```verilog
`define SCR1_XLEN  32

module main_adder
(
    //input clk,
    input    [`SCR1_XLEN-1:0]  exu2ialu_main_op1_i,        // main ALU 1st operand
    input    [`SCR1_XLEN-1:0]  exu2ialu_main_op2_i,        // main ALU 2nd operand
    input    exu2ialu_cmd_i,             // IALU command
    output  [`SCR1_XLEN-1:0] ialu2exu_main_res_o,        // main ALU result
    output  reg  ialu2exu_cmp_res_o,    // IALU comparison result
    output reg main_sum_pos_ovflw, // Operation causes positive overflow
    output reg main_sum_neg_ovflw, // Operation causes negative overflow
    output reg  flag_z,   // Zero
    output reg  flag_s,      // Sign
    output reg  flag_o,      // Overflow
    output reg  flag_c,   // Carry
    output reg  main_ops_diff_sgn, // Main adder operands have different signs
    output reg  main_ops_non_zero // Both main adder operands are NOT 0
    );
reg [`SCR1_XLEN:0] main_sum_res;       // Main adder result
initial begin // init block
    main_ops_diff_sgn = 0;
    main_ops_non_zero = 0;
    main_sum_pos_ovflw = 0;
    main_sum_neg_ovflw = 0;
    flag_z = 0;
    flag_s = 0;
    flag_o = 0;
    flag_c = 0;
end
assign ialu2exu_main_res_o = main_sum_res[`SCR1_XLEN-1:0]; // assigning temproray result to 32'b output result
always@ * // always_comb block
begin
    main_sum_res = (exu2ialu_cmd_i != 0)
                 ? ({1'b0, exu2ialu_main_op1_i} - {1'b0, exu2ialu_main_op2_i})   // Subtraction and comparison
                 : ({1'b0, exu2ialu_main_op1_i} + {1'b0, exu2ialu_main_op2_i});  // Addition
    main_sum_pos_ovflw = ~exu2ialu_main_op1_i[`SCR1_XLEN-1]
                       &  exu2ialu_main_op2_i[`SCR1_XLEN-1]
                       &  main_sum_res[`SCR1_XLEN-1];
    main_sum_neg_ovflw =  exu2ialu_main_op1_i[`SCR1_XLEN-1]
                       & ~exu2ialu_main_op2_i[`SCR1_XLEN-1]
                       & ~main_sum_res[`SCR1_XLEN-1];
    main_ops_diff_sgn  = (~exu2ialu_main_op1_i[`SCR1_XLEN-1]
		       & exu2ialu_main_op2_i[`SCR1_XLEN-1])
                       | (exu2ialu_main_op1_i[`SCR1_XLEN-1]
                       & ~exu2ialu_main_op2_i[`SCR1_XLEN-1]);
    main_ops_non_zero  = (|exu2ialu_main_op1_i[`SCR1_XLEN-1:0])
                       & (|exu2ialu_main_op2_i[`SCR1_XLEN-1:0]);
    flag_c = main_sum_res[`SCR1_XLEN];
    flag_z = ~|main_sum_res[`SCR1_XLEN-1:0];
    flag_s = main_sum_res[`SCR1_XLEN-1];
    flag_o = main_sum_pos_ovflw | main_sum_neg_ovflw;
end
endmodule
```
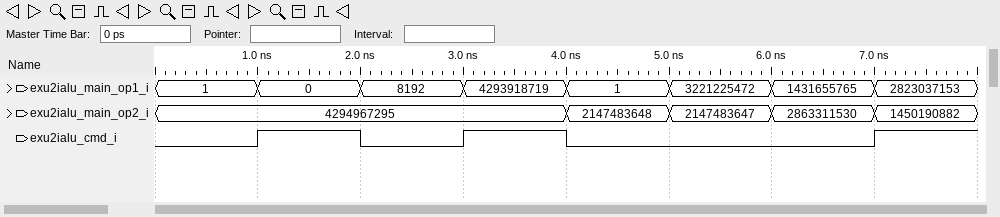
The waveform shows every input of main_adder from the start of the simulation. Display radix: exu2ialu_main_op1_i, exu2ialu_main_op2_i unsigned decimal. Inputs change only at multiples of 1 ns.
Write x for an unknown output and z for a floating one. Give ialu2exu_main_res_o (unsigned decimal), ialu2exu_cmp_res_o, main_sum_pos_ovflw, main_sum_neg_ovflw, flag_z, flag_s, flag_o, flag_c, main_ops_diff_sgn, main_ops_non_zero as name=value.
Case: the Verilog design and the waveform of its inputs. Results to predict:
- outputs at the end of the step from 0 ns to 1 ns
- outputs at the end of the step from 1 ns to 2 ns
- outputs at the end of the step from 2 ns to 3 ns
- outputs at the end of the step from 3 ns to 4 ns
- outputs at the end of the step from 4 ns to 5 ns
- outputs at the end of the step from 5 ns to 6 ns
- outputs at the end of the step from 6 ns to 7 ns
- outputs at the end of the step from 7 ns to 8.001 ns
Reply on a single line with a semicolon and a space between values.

ialu2exu_main_res_o=0, ialu2exu_cmp_res_o=x, main_sum_pos_ovflw=0, main_sum_neg_ovflw=0, flag_z=1, flag_s=0, flag_o=0, flag_c=1, main_ops_diff_sgn=1, main_ops_non_zero=1; ialu2exu_main_res_o=1, ialu2exu_cmp_res_o=x, main_sum_pos_ovflw=0, main_sum_neg_ovflw=0, flag_z=0, flag_s=0, flag_o=0, flag_c=1, main_ops_diff_sgn=1, main_ops_non_zero=0; ialu2exu_main_res_o=8191, ialu2exu_cmp_res_o=x, main_sum_pos_ovflw=0, main_sum_neg_ovflw=0, flag_z=0, flag_s=0, flag_o=0, flag_c=1, main_ops_diff_sgn=1, main_ops_non_zero=1; ialu2exu_main_res_o=4293918720, ialu2exu_cmp_res_o=x, main_sum_pos_ovflw=0, main_sum_neg_ovflw=0, flag_z=0, flag_s=1, flag_o=0, flag_c=1, main_ops_diff_sgn=0, main_ops_non_zero=1; ialu2exu_main_res_o=2147483649, ialu2exu_cmp_res_o=x, main_sum_pos_ovflw=1, main_sum_neg_ovflw=0, flag_z=0, flag_s=1, flag_o=1, flag_c=0, main_ops_diff_sgn=1, main_ops_non_zero=1; ialu2exu_main_res_o=1073741823, ialu2exu_cmp_res_o=x, main_sum_pos_ovflw=0, main_sum_neg_ovflw=1, flag_z=0, flag_s=0, flag_o=1, flag_c=1, main_ops_diff_sgn=1, main_ops_non_zero=1; ialu2exu_main_res_o=4294967295, ialu2exu_cmp_res_o=x, main_sum_pos_ovflw=1, main_sum_neg_ovflw=0, flag_z=0, flag_s=1, flag_o=1, flag_c=0, main_ops_diff_sgn=1, main_ops_non_zero=1; ialu2exu_main_res_o=1372846271, ialu2exu_cmp_res_o=x, main_sum_pos_ovflw=0, main_sum_neg_ovflw=1, flag_z=0, flag_s=0, flag_o=1, flag_c=0, main_ops_diff_sgn=1, main_ops_non_zero=1
